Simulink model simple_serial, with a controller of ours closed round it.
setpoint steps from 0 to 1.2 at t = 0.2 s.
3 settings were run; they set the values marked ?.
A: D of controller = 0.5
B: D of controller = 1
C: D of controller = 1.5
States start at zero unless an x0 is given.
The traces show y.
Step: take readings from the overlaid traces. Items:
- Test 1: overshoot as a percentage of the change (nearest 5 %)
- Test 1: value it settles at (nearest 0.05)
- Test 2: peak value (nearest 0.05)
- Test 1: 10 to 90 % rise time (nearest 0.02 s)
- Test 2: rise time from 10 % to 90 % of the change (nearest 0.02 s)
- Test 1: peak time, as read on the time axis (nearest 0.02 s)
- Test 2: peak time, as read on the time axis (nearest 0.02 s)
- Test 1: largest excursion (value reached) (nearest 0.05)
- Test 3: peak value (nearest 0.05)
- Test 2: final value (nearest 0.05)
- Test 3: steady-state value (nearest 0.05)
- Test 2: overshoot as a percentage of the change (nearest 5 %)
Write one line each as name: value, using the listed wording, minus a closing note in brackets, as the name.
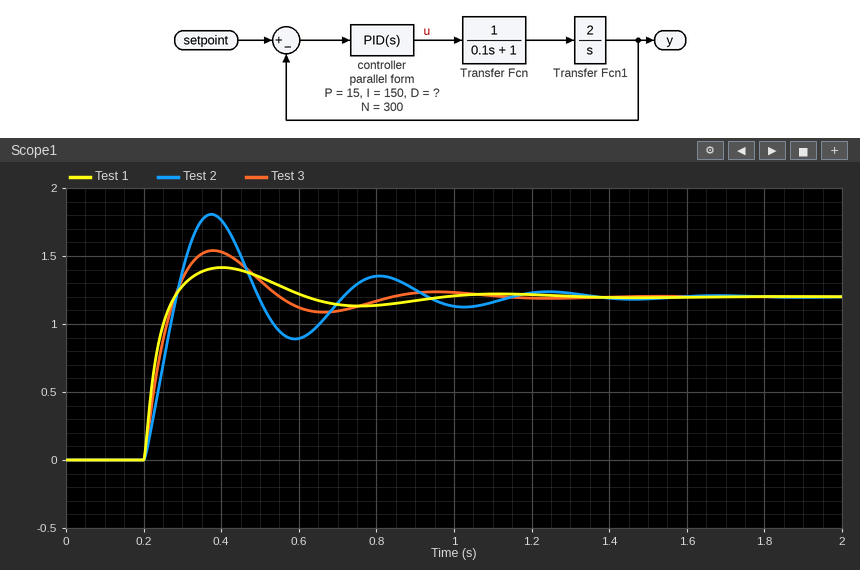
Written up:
Test 1: overshoot as a percentage of the change: 20 %
Test 1: value it settles at: 1.20
Test 2: peak value: 1.80
Test 1: 10 to 90 % rise time: 0.06 s
Test 2: rise time from 10 % to 90 % of the change: 0.06 s
Test 1: peak time, as read on the time axis: 0.40 s
Test 2: peak time, as read on the time axis: 0.38 s
Test 1: largest excursion (value reached): 1.40
Test 3: peak value: 1.55
Test 2: final value: 1.20
Test 3: steady-state value: 1.20
Test 2: overshoot as a percentage of the change: 50 %
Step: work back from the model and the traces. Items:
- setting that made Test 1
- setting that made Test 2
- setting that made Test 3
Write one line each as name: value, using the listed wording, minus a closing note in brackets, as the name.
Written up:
setting that made Test 1: C
setting that made Test 2: A
setting that made Test 3: B
